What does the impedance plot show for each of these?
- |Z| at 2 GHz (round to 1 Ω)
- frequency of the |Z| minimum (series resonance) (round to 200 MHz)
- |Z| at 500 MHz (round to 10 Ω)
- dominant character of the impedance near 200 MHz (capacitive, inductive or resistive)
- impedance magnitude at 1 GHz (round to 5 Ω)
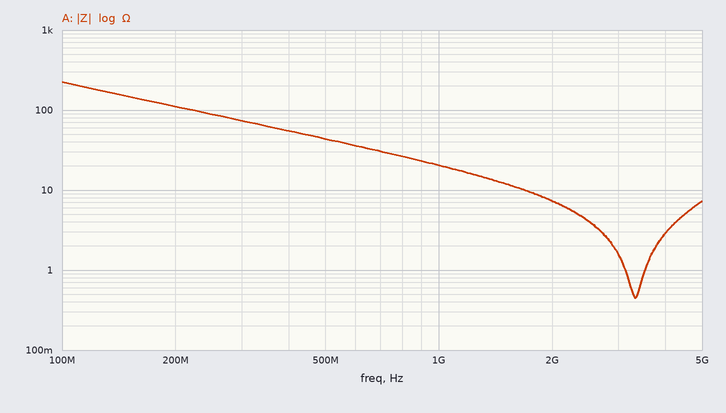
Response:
7 Ω
3.4 GHz
40 Ω
capacitive
20 Ω
